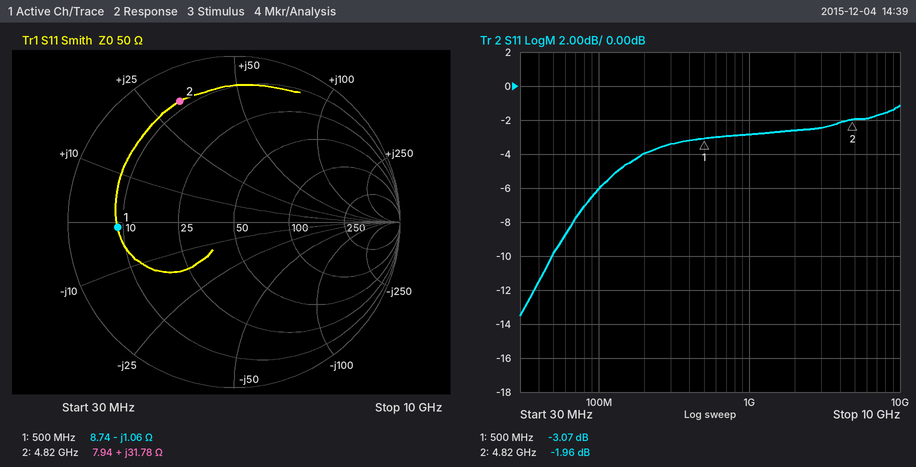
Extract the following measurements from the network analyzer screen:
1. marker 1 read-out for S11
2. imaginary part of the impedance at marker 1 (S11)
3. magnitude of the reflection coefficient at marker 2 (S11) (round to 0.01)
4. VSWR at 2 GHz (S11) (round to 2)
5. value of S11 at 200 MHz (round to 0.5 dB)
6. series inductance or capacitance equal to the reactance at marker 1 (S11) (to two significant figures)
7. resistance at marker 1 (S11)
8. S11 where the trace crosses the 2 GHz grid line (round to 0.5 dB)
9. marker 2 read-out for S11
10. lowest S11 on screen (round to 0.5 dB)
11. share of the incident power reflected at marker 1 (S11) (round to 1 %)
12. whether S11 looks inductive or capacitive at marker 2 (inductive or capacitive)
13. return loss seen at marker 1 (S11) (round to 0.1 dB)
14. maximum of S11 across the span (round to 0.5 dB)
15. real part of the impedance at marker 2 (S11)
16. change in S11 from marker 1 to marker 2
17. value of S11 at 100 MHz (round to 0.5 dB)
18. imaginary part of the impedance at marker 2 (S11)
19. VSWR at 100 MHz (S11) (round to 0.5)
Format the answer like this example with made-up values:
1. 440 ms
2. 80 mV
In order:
1. -3.07 dB
2. -1.06 Ω
3. 0.80
4. 6
5. -4.0 dB
6. 300 pF
7. 8.74 Ω
8. -2.5 dB
9. -1.96 dB
10. -13.5 dB
11. 49 %
12. inductive
13. 3.1 dB
14. -1.0 dB
15. 7.94 Ω
16. 1.11 dB
17. -6.0 dB
18. +31.78 Ω
19. 3.0
